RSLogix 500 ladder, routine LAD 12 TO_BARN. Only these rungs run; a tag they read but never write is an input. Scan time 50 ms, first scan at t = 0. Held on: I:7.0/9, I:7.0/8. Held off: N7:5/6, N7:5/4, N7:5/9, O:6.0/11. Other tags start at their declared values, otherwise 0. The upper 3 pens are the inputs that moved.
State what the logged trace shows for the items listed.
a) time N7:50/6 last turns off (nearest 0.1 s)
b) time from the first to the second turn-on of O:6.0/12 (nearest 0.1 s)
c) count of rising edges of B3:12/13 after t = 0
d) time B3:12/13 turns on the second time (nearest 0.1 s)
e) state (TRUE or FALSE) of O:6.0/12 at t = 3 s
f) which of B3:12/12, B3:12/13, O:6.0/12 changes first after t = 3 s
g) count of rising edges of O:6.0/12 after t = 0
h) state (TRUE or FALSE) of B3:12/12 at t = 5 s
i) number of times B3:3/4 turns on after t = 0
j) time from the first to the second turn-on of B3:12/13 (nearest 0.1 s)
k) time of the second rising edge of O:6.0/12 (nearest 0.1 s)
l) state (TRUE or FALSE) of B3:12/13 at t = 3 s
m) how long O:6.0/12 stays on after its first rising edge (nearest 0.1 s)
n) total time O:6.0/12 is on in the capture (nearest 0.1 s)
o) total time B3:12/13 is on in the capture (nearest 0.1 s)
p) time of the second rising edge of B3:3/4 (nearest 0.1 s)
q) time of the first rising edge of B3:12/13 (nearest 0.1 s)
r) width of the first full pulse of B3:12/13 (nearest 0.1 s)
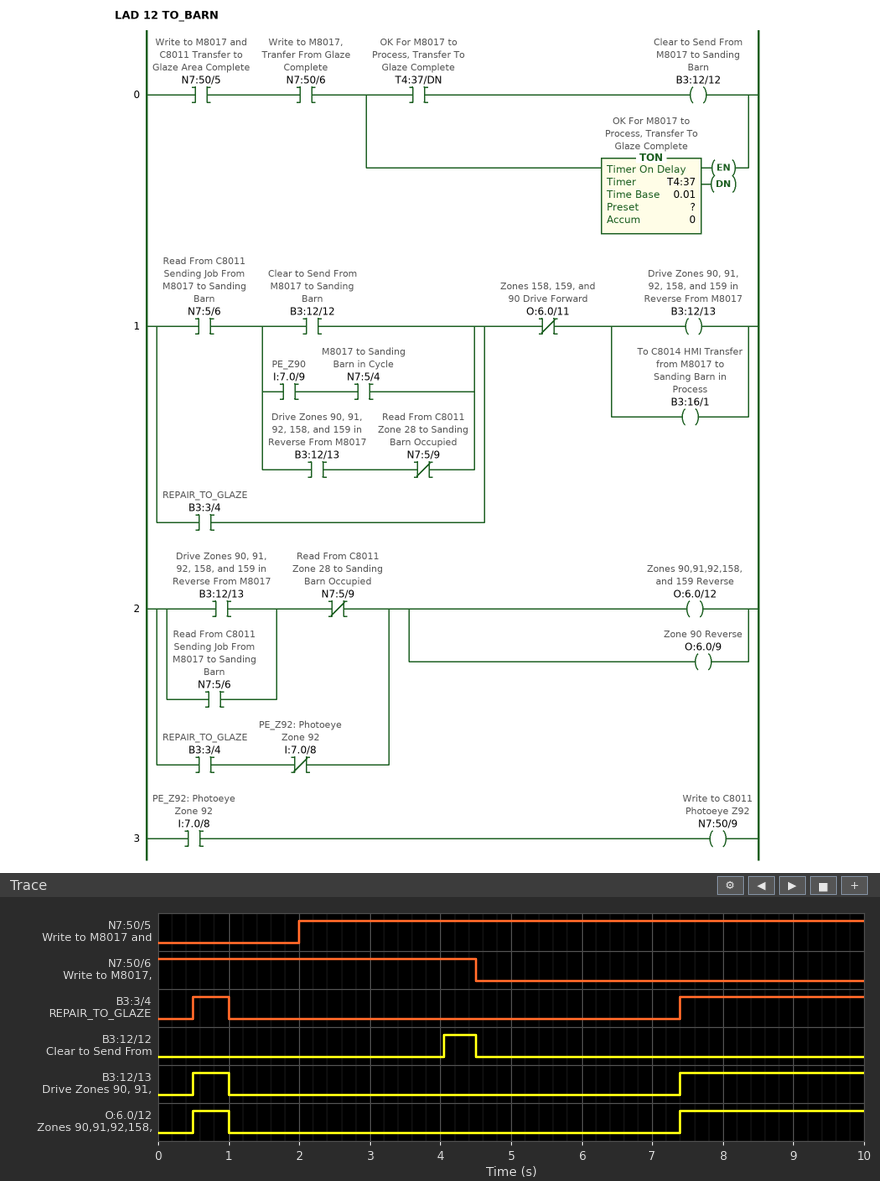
4.5 s
6.9 s
2
7.4 s
FALSE
B3:12/12
2
FALSE
2
6.9 s
7.4 s
FALSE
0.5 s
3.1 s
3.1 s
7.4 s
0.5 s
0.5 s
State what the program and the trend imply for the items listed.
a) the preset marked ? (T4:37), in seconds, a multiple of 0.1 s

2.0 s
